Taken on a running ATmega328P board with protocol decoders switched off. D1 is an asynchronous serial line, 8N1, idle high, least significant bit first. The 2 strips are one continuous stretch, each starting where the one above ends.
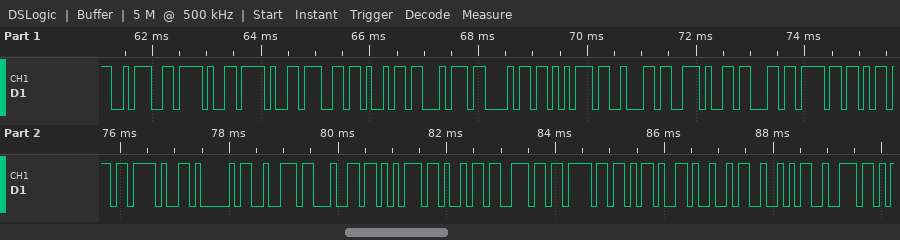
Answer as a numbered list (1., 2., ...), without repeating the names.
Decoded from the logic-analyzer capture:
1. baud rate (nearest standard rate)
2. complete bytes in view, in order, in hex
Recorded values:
1. 9600 baud
2. 3A 2F 2F 67 69 74 68 75 62 2E 63 6F 6D 2F 41 72 64 75 69 6E 6F 2D 49 52 72
